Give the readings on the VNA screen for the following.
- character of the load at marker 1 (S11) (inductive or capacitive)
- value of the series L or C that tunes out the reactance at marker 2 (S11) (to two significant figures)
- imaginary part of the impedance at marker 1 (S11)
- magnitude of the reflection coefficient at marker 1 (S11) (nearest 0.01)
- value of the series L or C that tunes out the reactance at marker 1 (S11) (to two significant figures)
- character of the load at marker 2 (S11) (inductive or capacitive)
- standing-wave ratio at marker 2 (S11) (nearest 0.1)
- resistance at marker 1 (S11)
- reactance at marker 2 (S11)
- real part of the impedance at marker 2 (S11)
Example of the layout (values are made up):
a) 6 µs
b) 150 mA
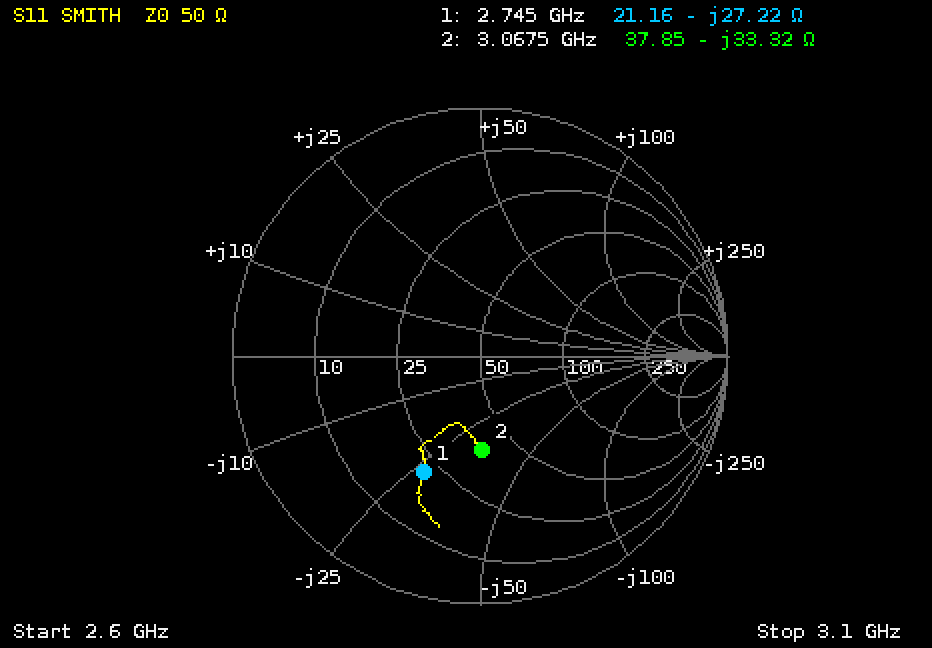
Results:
a) capacitive
b) 1.7 nH
c) -27.22 Ω
d) 0.52
e) 1.6 nH
f) capacitive
g) 2.2
h) 21.16 Ω
i) -33.32 Ω
j) 37.85 Ω
